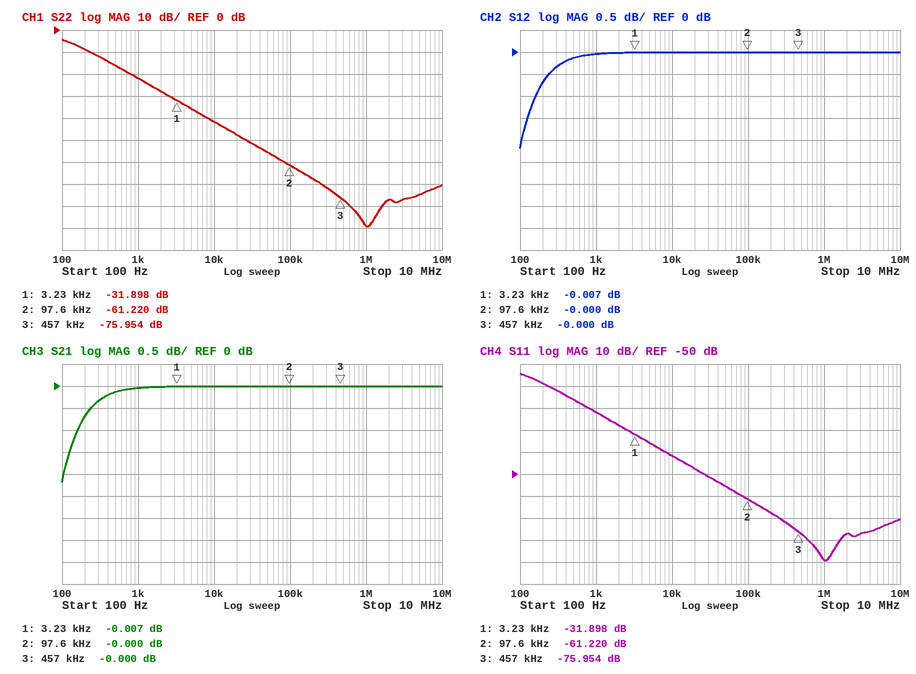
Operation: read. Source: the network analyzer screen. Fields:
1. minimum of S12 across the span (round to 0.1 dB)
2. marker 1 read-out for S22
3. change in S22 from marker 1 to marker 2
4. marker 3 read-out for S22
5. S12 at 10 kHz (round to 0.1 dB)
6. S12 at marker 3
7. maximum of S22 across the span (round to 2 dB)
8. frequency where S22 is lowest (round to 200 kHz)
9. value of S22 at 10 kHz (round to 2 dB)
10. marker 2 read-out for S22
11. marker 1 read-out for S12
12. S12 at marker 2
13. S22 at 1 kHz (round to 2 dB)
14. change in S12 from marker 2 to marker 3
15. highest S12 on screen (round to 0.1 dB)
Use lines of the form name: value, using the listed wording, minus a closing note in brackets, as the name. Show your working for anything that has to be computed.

minimum of S12 across the span: -2.2 dB
marker 1 read-out for S22: -31.898 dB
change in S22 from marker 1 to marker 2: -61.22 − (-31.898) = -29.322 dB
marker 3 read-out for S22: -75.954 dB
S12 at 10 kHz: 0.0 dB
S12 at marker 3: -0.000 dB
maximum of S22 across the span: -4 dB
frequency where S22 is lowest: 1.0 MHz
value of S22 at 10 kHz: -42 dB
marker 2 read-out for S22: -61.220 dB
marker 1 read-out for S12: -0.007 dB
S12 at marker 2: -0.000 dB
S22 at 1 kHz: -22 dB
change in S12 from marker 2 to marker 3: -0 − (-0) = 0.000 dB
highest S12 on screen: 0.0 dB
